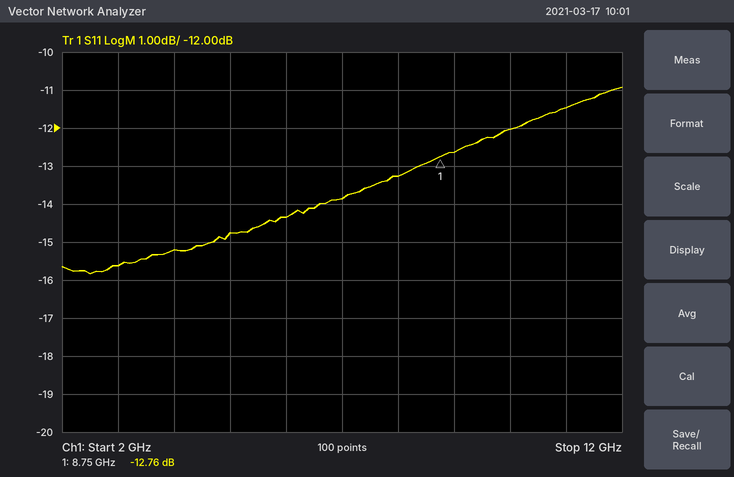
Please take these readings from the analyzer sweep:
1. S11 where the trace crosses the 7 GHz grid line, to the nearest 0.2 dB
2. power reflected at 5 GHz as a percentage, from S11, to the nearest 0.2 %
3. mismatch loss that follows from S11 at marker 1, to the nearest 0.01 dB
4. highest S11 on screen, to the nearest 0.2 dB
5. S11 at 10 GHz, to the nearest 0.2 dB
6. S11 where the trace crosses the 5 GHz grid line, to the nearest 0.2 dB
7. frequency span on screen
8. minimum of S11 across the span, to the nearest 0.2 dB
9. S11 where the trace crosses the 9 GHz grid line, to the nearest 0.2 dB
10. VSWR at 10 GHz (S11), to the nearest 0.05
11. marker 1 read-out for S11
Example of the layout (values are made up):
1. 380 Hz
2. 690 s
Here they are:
1. -13.8 dB
2. 3.4 %
3. 0.24 dB
4. -11.0 dB
5. -12.0 dB
6. -14.8 dB
7. 10 GHz
8. -15.8 dB
9. -12.6 dB
10. 1.65
11. -12.76 dB
